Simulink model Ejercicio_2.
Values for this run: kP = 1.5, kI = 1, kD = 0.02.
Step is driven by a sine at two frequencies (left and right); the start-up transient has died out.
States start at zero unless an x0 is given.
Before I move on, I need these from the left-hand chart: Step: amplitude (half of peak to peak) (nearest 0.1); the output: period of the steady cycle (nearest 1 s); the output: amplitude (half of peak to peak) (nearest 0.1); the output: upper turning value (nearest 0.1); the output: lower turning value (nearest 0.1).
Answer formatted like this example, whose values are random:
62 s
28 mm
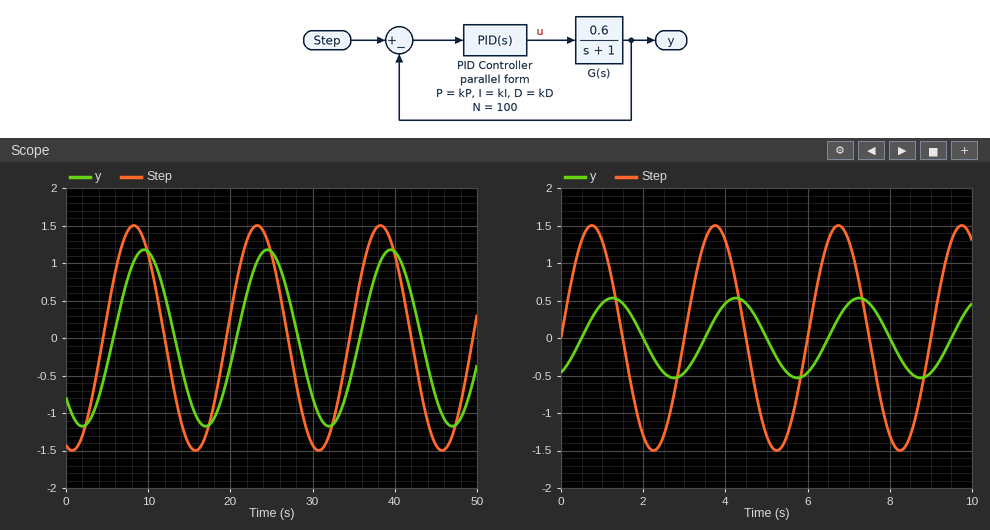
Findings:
1.5
15 s
1.2
1.2
-1.2
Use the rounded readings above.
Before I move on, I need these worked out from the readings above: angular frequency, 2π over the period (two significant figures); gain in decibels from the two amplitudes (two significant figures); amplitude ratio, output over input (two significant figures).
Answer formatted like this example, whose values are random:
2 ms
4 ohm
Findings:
0.42 rad/s
-1.9 dB
0.80
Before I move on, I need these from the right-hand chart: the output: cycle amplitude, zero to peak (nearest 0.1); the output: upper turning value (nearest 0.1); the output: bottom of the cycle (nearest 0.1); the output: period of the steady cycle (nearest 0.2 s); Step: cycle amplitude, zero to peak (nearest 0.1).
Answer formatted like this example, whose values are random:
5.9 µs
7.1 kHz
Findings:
0.5
0.5
-0.5
3.0 s
1.5
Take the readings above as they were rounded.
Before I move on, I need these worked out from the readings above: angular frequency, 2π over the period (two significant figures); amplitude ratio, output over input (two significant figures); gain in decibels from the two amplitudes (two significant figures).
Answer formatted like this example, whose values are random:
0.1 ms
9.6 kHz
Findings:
2.1 rad/s
0.33
-9.5 dB
